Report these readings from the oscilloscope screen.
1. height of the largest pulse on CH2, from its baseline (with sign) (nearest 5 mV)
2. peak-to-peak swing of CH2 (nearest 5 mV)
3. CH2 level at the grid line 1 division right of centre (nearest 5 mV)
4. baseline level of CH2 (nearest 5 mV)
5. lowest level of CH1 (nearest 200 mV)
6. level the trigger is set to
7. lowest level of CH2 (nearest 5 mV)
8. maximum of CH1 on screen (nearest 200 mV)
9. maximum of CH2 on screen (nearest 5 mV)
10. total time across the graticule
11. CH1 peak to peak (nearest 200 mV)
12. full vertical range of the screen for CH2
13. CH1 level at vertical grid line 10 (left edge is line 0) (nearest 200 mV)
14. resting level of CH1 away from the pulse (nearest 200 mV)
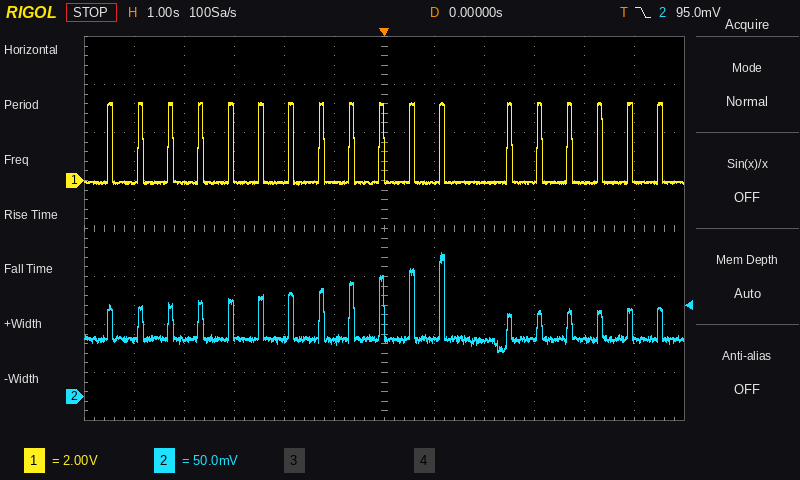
+90 mV
105 mV
60 mV
60 mV
-200 mV
95.0 mV
45 mV
3.2 V
150 mV
12 s
3.4 V
400 mV
0.0 V
0.0 V
